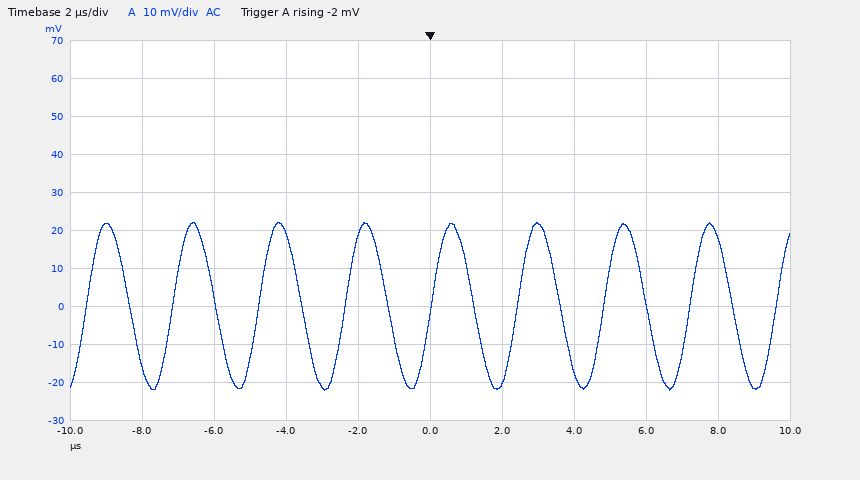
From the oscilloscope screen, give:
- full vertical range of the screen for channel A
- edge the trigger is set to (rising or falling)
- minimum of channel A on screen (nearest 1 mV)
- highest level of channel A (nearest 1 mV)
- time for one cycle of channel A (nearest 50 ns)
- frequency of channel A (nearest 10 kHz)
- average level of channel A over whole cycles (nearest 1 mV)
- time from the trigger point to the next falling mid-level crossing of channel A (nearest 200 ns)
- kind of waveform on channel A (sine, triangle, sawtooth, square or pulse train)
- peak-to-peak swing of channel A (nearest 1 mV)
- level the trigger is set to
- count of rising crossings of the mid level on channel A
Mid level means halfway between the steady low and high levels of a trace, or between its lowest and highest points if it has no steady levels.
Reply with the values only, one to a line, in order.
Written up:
100 mV
rising
-22 mV
22 mV
2.40 µs
420 kHz
0 mV
1.2 µs
sine
44 mV
-2 mV
9
